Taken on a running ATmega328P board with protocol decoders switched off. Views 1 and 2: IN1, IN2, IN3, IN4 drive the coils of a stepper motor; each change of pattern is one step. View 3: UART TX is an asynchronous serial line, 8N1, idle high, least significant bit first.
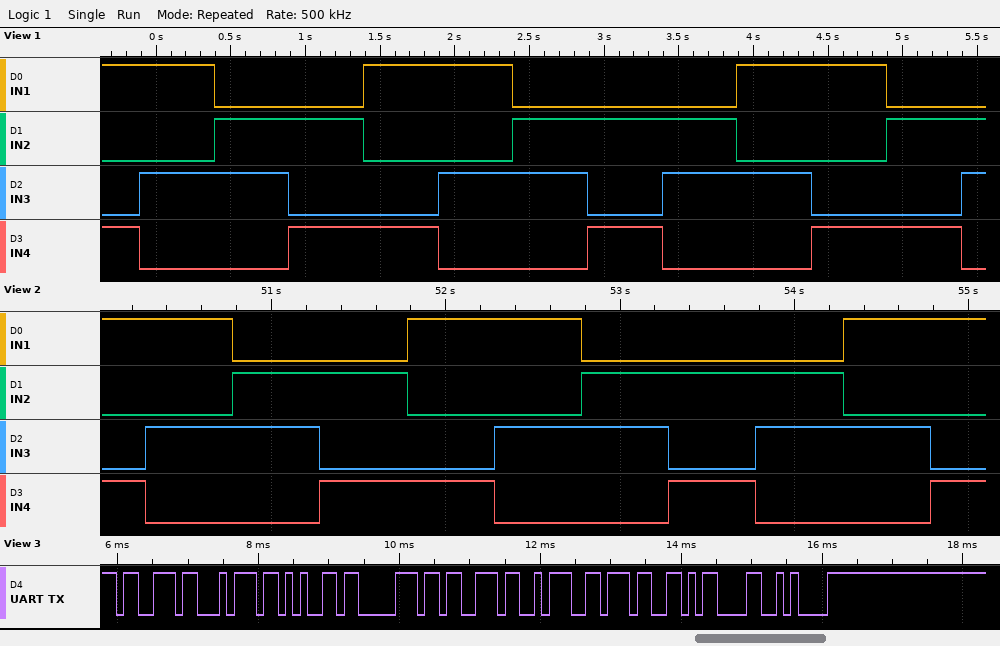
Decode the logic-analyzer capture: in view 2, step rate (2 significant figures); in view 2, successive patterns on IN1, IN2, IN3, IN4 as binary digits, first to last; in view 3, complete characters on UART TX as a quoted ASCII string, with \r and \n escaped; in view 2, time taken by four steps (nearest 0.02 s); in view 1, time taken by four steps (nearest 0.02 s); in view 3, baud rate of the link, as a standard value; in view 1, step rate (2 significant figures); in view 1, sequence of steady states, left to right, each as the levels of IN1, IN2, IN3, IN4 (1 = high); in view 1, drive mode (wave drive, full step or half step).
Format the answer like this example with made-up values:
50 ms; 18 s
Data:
2.0 steps/s; 1001 1010 0110 0101 1001 1010 0110 0101 0110 1010 1001; "steps:7\r\n"; 2.00 s; 2.00 s; 9600 baud; 2.0 steps/s; 1001 1010 0110 0101 1001 1010 0110 0101 0110 1010 1001 0101 0110; full step
